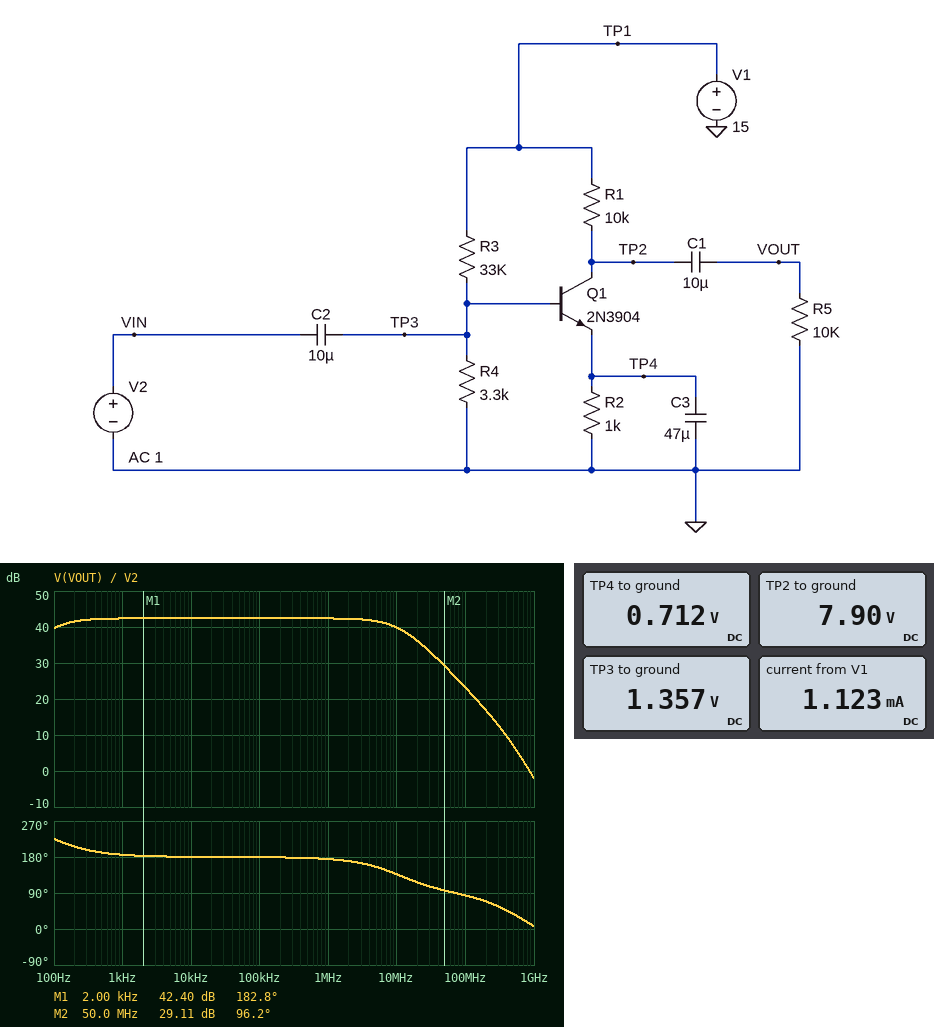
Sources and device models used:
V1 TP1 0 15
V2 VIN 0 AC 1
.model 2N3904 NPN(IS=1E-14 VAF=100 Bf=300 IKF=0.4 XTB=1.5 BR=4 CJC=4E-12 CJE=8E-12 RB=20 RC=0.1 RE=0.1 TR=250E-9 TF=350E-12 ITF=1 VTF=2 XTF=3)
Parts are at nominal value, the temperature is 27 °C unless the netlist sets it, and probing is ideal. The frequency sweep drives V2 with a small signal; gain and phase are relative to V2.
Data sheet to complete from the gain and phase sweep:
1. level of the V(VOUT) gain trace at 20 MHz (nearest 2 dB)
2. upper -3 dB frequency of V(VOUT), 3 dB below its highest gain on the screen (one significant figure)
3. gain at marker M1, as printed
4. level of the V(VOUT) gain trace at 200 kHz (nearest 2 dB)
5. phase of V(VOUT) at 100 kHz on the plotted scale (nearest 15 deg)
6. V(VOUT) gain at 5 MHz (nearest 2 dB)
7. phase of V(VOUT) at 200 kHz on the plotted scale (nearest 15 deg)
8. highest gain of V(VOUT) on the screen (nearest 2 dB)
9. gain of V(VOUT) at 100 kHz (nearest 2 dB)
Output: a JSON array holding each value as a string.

["36 dB", "10 MHz", "42.40 dB", "42 dB", "180 deg", "42 dB", "180 deg", "42 dB", "42 dB"]
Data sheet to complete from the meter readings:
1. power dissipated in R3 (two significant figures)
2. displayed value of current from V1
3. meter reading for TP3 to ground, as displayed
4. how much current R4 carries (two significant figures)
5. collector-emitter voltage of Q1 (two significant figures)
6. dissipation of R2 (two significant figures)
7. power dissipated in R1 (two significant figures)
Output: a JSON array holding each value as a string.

["5.6 mW", "1.123 mA", "1.357 V", "410 µA", "7.2 V", "510 µW", "5.0 mW"]
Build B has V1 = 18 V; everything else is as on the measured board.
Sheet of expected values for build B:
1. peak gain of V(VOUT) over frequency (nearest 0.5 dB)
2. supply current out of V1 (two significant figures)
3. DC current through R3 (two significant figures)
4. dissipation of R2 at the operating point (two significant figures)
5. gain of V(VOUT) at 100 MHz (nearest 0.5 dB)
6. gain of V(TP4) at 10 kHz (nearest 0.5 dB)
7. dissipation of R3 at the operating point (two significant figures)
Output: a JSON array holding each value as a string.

["45.0 dB", "1.5 mA", "500 µA", "950 µW", "25.0 dB", "-38.5 dB", "8.1 mW"]
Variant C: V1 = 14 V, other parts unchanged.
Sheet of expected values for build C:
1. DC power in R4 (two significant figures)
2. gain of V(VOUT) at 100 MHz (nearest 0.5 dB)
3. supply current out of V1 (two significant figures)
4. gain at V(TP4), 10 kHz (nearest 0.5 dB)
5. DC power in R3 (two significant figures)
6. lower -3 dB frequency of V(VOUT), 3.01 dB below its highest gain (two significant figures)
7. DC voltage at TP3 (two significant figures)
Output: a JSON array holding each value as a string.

["490 µW", "22.5 dB", "1.0 mA", "-42.0 dB", "4.9 mW", "84 Hz", "1.3 V"]
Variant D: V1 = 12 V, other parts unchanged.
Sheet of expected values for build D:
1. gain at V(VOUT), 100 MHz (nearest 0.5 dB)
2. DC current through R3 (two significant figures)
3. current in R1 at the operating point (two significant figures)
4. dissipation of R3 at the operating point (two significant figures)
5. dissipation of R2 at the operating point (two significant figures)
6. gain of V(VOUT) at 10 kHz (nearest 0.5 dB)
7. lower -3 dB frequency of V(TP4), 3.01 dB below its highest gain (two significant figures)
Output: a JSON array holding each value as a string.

["20.5 dB", "330 µA", "450 µA", "3.6 mW", "210 µW", "38.5 dB", "4.6 Hz"]
